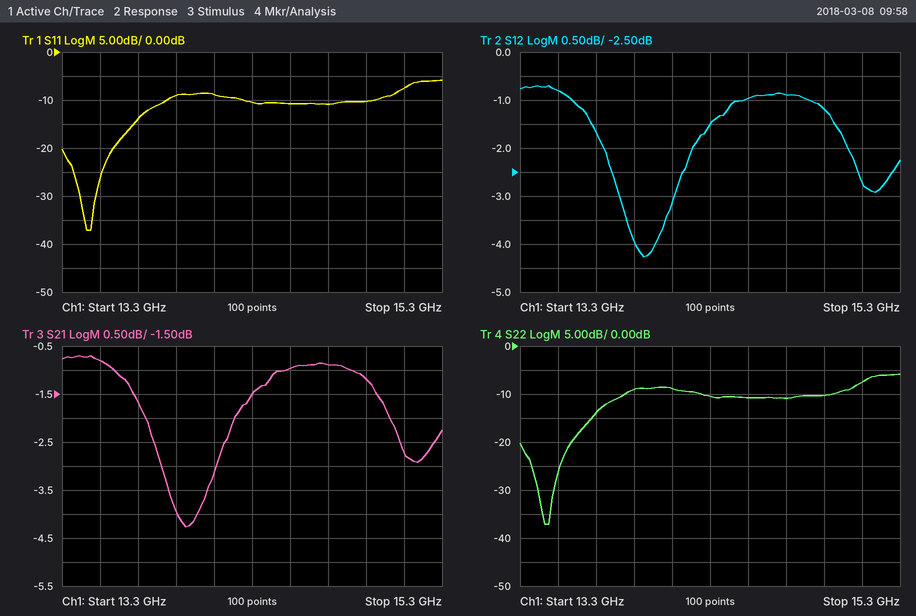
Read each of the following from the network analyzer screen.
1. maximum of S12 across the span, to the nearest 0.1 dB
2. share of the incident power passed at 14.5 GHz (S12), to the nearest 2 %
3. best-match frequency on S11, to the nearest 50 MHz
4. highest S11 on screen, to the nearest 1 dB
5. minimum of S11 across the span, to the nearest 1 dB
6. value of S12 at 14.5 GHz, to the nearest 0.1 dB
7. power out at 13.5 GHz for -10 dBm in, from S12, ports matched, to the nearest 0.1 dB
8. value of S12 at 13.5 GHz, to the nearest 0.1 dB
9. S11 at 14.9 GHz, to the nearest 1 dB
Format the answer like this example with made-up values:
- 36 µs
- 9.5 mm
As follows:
- -0.7 dB
- 80 %
- 13.45 GHz
- -6 dB
- -37 dB
- -1.0 dB
- -10.8 dBm
- -0.8 dB
- -10 dB
